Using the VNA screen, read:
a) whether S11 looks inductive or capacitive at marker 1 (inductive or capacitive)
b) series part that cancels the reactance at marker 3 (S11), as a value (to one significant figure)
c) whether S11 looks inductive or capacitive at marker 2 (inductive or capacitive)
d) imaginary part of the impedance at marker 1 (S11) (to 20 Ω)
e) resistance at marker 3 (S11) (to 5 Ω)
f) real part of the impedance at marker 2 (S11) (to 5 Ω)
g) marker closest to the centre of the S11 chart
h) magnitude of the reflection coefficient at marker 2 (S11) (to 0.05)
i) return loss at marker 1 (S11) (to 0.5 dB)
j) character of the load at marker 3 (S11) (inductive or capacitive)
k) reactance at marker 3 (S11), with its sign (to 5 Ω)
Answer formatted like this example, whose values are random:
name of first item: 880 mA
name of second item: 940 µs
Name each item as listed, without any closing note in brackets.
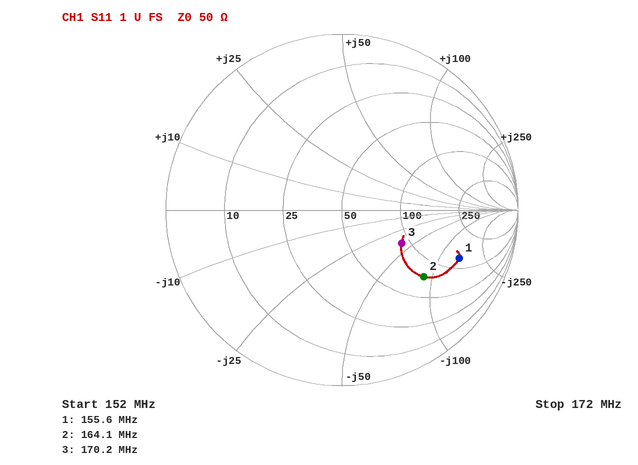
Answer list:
whether S11 looks inductive or capacitive at marker 1: capacitive
series part that cancels the reactance at marker 3 (S11), as a value: 40 nH
whether S11 looks inductive or capacitive at marker 2: capacitive
imaginary part of the impedance at marker 1 (S11): -140 Ω
resistance at marker 3 (S11): 90 Ω
real part of the impedance at marker 2 (S11): 75 Ω
marker closest to the centre of the S11 chart: marker 3
magnitude of the reflection coefficient at marker 2 (S11): 0.60
return loss at marker 1 (S11): 3.0 dB
character of the load at marker 3 (S11): capacitive
reactance at marker 3 (S11), with its sign: -40 Ω
